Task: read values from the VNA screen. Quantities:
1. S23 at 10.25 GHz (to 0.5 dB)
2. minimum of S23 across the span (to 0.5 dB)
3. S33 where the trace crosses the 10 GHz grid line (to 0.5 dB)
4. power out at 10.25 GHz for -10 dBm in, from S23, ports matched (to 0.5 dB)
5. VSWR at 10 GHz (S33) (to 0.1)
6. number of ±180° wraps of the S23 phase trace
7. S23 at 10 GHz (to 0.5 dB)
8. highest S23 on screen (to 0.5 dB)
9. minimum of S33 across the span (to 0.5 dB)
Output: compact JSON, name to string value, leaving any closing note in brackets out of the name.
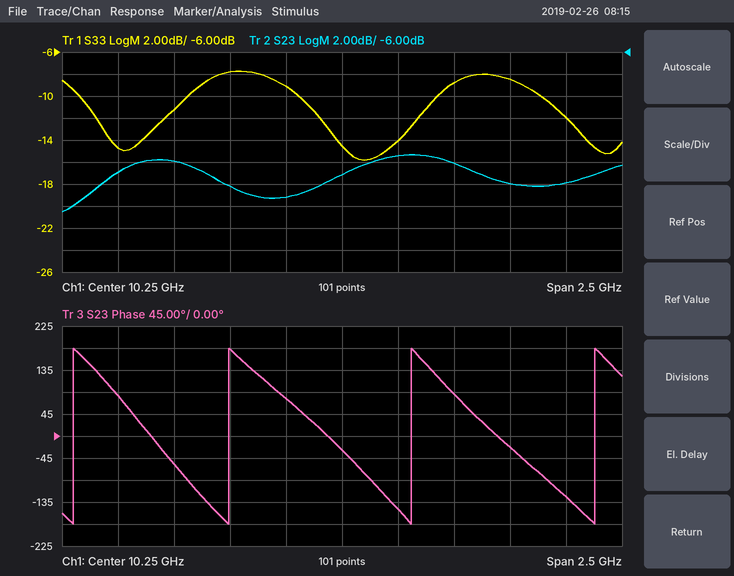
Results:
{"S23 at 10.25 GHz": "-17.0 dB", "minimum of S23 across the span": "-20.5 dB", "S33 where the trace crosses the 10 GHz grid line": "-9.0 dB", "power out at 10.25 GHz for -10 dBm in, from S23, ports matched": "-27.0 dBm", "VSWR at 10 GHz (S33)": "2.1", "number of ±180° wraps of the S23 phase trace": "4", "S23 at 10 GHz": "-19.0 dB", "highest S23 on screen": "-15.5 dB", "minimum of S33 across the span": "-16.0 dB"}
